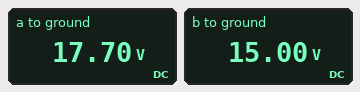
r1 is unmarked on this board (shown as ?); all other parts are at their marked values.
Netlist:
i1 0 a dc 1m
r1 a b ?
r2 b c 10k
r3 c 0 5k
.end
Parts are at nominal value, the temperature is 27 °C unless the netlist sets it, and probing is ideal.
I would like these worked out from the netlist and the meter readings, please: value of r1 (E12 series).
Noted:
2.7 kΩ
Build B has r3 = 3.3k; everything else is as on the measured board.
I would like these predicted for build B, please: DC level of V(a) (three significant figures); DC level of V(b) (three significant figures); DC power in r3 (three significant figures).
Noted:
16.0 V
13.3 V
3.30 mW
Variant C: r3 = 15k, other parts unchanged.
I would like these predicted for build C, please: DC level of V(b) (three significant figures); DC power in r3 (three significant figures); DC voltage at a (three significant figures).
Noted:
25.0 V
15.0 mW
27.7 V
